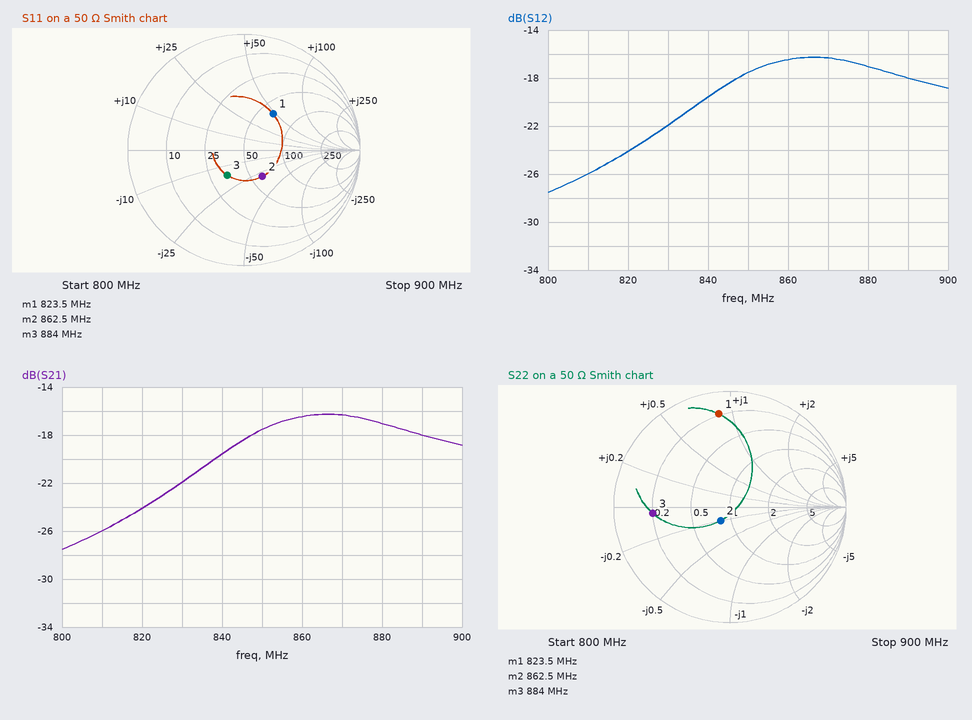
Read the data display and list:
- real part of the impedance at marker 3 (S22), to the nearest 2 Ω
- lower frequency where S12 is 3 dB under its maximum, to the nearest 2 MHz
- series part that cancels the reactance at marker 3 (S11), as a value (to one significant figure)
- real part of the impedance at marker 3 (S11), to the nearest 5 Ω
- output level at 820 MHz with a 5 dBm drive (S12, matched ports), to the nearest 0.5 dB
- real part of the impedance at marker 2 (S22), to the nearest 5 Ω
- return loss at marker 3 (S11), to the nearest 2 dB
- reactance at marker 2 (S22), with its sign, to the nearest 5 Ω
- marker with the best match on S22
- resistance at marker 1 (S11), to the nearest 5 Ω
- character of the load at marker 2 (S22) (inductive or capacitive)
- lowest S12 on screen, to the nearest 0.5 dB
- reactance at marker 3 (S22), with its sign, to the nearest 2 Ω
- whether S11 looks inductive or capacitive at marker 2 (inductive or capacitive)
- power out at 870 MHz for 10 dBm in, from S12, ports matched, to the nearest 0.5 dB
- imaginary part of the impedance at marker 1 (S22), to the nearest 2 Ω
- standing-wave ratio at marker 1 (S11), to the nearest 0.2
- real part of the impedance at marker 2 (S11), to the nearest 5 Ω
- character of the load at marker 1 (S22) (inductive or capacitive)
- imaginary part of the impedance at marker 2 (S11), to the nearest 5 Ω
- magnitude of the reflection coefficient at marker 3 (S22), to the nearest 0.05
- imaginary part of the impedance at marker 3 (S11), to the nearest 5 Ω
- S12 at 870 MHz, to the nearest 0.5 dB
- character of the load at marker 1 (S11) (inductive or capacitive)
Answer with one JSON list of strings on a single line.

["10 Ω", "842 MHz", "3 nH", "35 Ω", "-19.0 dBm", "40 Ω", "12 dB", "-10 Ω", "marker 2", "65 Ω", "capacitive", "-27.5 dB", "-2 Ω", "capacitive", "-6.5 dBm", "+44 Ω", "2.4", "60 Ω", "inductive", "-30 Ω", "0.65", "-15 Ω", "-16.5 dB", "inductive"]
